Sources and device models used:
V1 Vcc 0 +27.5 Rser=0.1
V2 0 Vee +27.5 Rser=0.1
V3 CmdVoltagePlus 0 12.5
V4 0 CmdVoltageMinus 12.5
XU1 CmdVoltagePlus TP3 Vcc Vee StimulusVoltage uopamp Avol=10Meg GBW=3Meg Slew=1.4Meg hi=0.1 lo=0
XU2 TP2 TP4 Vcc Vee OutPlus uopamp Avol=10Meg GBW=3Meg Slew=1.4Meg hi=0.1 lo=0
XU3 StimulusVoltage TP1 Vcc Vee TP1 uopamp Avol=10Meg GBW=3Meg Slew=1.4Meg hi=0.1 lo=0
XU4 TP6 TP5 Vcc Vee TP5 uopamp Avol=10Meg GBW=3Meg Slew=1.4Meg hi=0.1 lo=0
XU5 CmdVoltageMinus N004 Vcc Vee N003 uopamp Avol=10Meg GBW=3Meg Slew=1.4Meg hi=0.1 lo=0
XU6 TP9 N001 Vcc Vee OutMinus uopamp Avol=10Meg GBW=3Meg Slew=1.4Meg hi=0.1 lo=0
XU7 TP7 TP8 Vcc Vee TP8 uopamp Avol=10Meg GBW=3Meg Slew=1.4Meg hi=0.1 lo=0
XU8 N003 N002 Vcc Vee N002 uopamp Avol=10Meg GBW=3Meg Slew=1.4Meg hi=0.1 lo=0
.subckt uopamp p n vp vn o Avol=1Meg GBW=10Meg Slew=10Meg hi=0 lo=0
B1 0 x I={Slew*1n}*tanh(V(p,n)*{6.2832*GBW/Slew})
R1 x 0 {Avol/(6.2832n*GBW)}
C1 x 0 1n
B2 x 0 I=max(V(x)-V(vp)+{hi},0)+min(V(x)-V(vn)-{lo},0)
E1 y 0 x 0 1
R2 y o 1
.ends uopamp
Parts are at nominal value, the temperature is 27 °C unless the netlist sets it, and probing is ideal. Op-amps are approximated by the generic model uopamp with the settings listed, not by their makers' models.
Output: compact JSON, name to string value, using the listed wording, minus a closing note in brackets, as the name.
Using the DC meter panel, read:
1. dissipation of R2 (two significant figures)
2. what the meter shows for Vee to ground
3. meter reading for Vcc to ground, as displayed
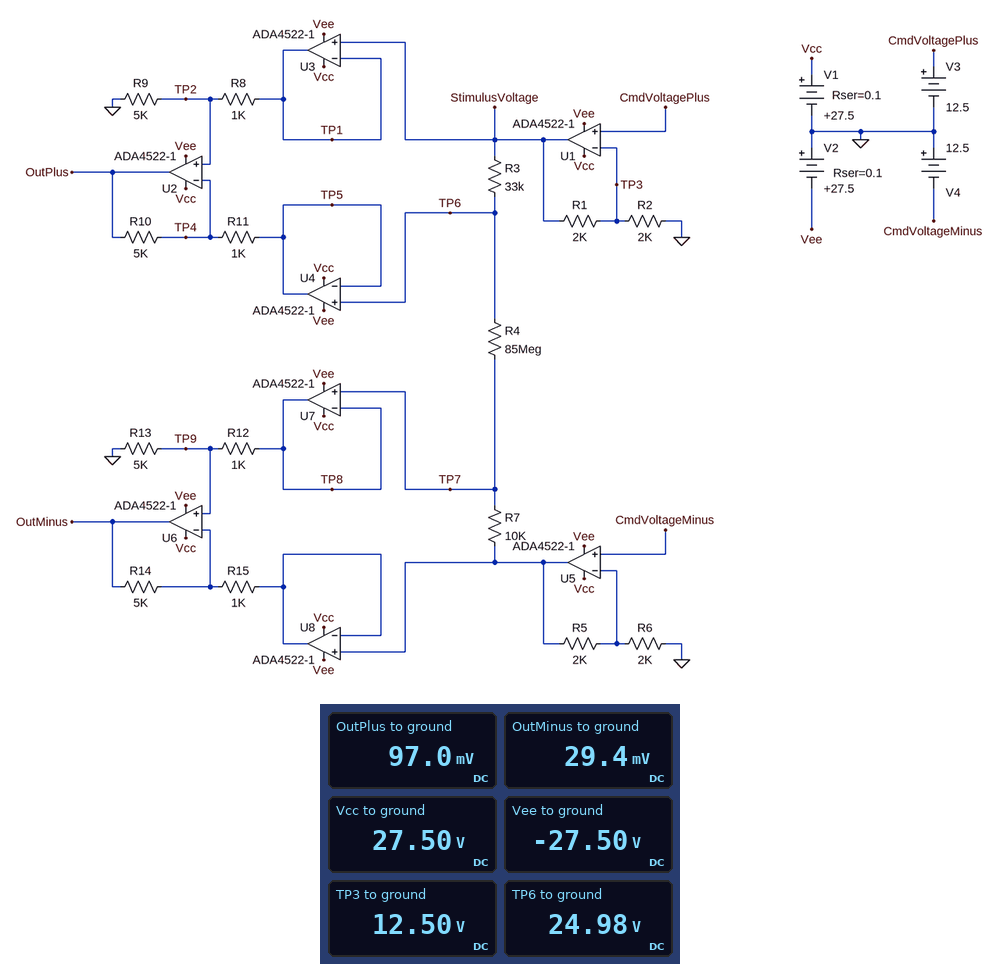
{"dissipation of R2": "78 mW", "what the meter shows for Vee to ground": "-27.50 V", "meter reading for Vcc to ground, as displayed": "27.50 V"}
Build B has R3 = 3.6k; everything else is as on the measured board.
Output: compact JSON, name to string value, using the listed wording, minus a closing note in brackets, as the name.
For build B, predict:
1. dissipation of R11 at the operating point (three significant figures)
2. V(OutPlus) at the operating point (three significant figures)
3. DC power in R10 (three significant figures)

{"dissipation of R11 at the operating point": "17.3 mW", "V(OutPlus) at the operating point": "10.6 mV", "DC power in R10": "86.7 mW"}
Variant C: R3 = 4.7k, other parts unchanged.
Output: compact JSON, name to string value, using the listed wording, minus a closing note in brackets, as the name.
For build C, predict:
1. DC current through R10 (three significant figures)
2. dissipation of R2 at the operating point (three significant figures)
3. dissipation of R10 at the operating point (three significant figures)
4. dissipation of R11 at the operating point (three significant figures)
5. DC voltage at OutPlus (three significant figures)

{"DC current through R10": "4.16 mA", "dissipation of R2 at the operating point": "78.1 mW", "dissipation of R10 at the operating point": "86.7 mW", "dissipation of R11 at the operating point": "17.3 mW", "DC voltage at OutPlus": "13.8 mV"}
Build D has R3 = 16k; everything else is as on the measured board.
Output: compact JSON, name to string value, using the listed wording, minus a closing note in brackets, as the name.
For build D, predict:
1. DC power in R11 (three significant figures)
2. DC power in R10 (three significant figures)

{"DC power in R11": "17.3 mW", "DC power in R10": "86.4 mW"}
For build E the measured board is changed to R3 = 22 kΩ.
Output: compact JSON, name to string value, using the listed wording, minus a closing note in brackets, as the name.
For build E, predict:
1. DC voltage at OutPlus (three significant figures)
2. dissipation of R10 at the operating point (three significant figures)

{"DC voltage at OutPlus": "64.7 mV", "dissipation of R10 at the operating point": "86.3 mW"}
